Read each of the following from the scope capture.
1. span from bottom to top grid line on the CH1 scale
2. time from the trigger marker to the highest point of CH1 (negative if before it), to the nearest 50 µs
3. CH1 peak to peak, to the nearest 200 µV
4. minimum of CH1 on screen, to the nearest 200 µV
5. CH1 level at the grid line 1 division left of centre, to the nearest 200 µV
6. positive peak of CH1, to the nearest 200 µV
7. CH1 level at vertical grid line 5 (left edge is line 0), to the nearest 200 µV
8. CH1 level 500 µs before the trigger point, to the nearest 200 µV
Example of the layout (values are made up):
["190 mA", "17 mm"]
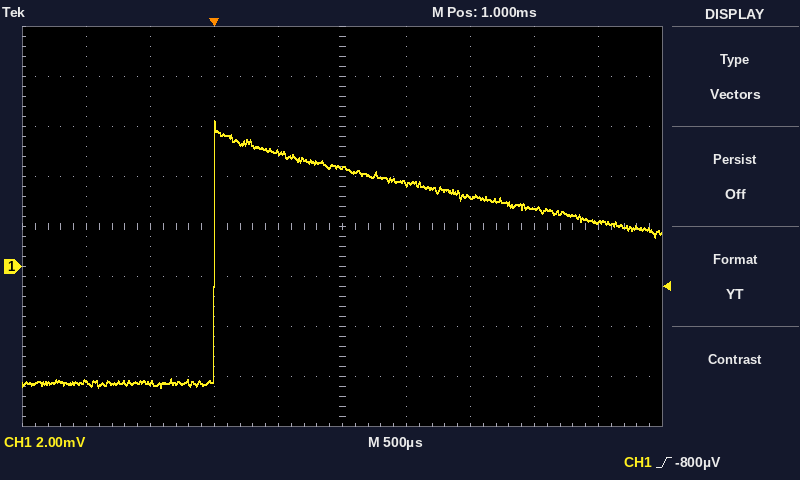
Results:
["16 mV", "0 µs", "10.6 mV", "-4.8 mV", "4.6 mV", "5.8 mV", "4.0 mV", "-4.6 mV"]
